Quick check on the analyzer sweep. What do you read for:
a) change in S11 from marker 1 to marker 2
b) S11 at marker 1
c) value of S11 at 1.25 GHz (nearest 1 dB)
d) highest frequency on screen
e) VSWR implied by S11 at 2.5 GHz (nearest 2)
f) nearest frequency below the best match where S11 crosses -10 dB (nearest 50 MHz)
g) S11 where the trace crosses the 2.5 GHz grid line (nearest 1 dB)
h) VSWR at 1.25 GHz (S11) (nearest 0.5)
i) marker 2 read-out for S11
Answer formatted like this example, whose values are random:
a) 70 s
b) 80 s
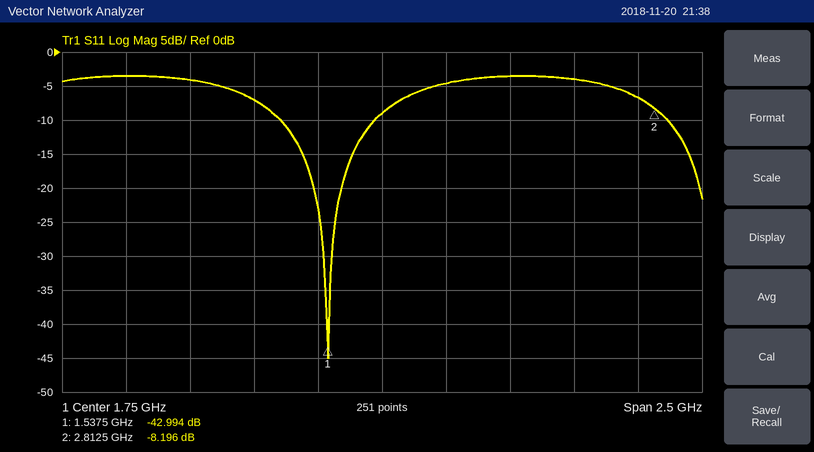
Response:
a) 34.798 dB
b) -42.994 dB
c) -7 dB
d) 3 GHz
e) 4
f) 1.35 GHz
g) -4 dB
h) 2.5
i) -8.196 dB
